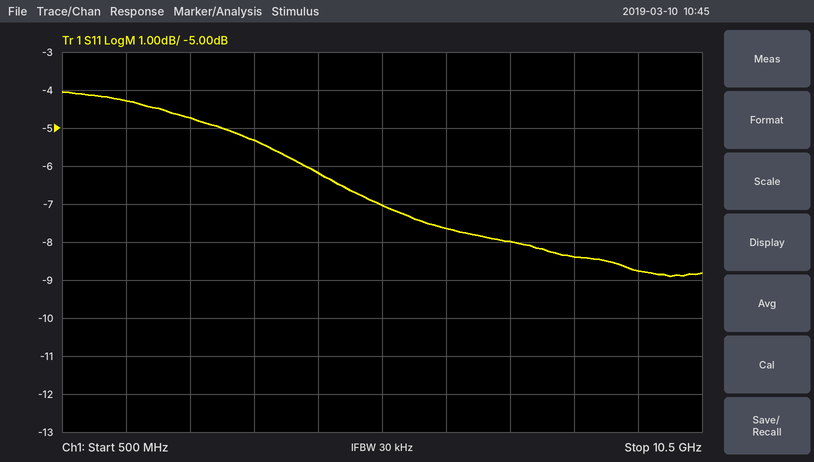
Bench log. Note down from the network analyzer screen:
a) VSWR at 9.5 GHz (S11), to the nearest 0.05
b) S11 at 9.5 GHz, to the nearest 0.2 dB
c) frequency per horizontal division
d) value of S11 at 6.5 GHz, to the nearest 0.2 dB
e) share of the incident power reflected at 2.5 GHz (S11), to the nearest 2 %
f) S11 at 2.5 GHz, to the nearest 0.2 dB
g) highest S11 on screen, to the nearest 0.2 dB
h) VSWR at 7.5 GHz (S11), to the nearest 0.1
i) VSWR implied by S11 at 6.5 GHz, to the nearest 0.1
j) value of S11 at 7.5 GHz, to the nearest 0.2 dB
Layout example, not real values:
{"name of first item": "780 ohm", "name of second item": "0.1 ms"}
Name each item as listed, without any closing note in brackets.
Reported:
{"VSWR at 9.5 GHz (S11), to the nearest 0.05": "2.15", "S11 at 9.5 GHz, to the nearest 0.2 dB": "-8.8 dB", "frequency per horizontal division": "1 GHz", "value of S11 at 6.5 GHz, to the nearest 0.2 dB": "-7.6 dB", "share of the incident power reflected at 2.5 GHz (S11), to the nearest 2 %": "34 %", "S11 at 2.5 GHz, to the nearest 0.2 dB": "-4.8 dB", "highest S11 on screen, to the nearest 0.2 dB": "-4.0 dB", "VSWR at 7.5 GHz (S11), to the nearest 0.1": "2.3", "VSWR implied by S11 at 6.5 GHz, to the nearest 0.1": "2.4", "value of S11 at 7.5 GHz, to the nearest 0.2 dB": "-8.0 dB"}
